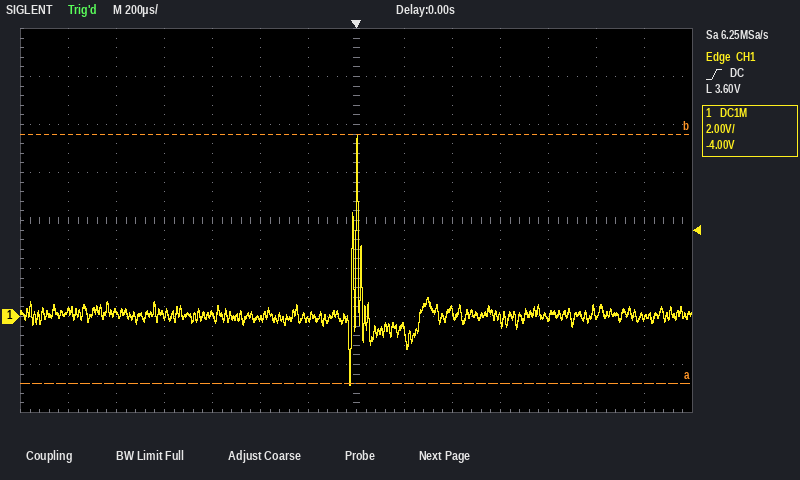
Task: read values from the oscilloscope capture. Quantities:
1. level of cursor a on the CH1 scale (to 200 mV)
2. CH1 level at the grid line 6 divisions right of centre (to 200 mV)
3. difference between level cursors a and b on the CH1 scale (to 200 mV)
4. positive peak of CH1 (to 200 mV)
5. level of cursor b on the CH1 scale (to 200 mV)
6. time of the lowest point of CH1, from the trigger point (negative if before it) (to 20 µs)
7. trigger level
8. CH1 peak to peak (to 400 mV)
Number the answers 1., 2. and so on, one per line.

1. -2.8 V
2. 0.0 V
3. 10.4 V
4. 7.6 V
5. 7.6 V
6. -20 µs
7. 3.60 V
8. 10.4 V
